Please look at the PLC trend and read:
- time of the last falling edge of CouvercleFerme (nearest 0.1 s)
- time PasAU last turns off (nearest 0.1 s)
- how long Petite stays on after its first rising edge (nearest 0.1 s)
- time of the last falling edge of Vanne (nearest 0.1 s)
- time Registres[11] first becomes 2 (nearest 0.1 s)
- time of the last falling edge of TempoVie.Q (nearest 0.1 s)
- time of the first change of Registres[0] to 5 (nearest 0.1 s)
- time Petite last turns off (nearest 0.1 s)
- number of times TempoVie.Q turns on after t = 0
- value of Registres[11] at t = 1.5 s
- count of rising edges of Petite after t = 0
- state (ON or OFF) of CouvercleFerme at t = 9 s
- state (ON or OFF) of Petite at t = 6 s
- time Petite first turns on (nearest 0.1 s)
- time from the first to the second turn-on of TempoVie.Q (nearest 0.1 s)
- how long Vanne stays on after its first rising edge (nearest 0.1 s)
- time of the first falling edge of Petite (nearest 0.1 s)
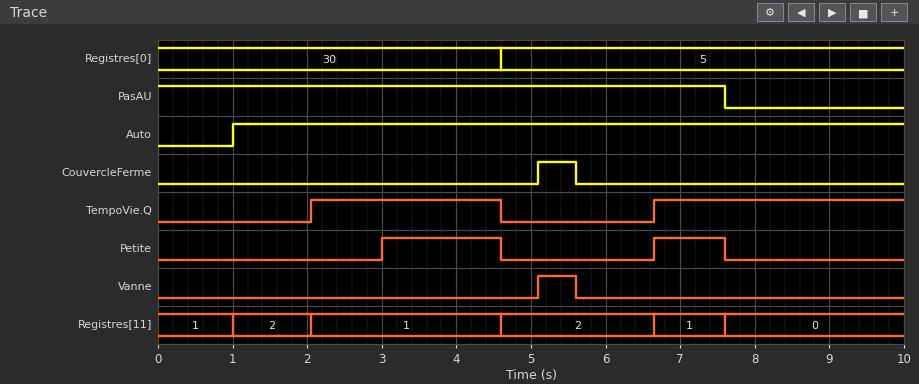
5.6 s
7.6 s
1.6 s
5.6 s
1.0 s
4.6 s
4.6 s
7.6 s
2
2
2
OFF
OFF
3.0 s
4.6 s
0.5 s
4.6 s
